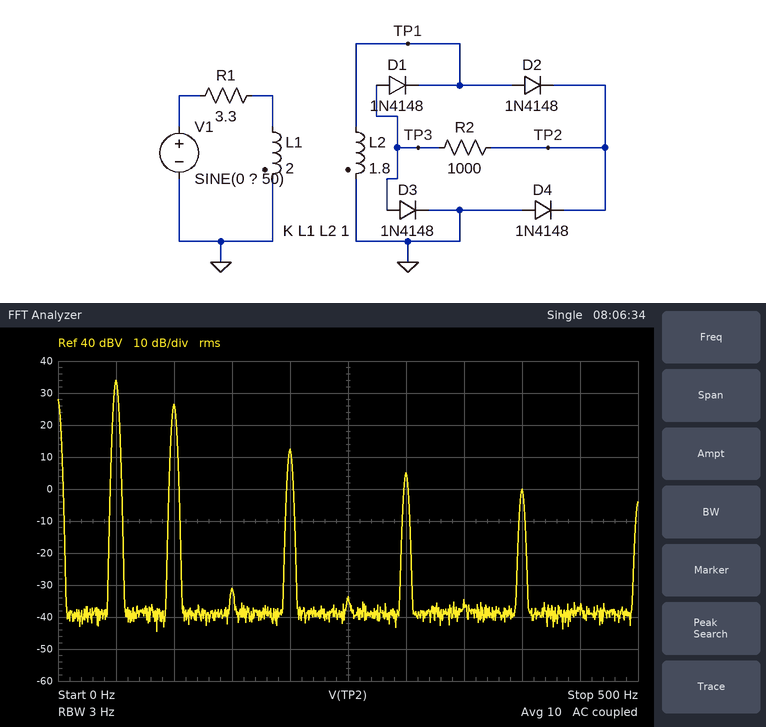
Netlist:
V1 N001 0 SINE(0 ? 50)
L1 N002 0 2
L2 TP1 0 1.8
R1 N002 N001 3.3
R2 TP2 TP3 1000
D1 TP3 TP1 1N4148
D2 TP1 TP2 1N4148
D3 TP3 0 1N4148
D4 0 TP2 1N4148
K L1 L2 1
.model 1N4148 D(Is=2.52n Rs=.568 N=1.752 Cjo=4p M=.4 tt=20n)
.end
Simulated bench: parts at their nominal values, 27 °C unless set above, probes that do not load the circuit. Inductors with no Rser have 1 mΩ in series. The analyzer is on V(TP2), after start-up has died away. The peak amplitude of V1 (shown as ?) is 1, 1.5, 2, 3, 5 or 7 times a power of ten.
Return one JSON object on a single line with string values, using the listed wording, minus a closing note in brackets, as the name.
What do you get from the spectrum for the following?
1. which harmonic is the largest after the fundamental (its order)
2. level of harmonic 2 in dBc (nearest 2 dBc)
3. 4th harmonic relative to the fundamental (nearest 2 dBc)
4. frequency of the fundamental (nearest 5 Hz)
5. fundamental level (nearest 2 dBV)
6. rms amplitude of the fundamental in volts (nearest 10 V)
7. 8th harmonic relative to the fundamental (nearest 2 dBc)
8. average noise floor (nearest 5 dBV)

{"which harmonic is the largest after the fundamental": "2", "level of harmonic 2 in dBc": "-8 dBc", "4th harmonic relative to the fundamental": "-22 dBc", "frequency of the fundamental": "50 Hz", "fundamental level": "34 dBV", "rms amplitude of the fundamental in volts": "50 V", "8th harmonic relative to the fundamental": "-34 dBc", "average noise floor": "-40 dBV"}
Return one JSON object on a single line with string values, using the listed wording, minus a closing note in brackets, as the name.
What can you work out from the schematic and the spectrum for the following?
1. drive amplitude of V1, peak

{"drive amplitude of V1, peak": "150 V"}
